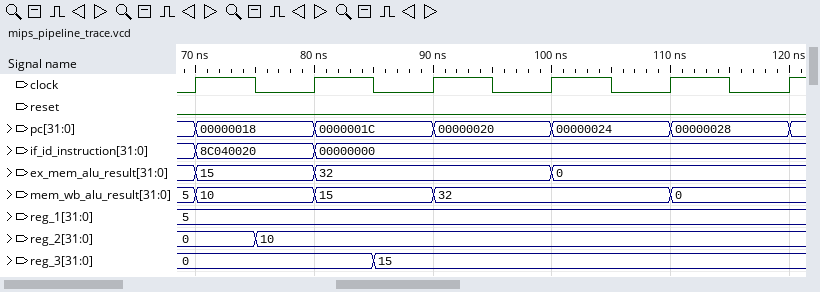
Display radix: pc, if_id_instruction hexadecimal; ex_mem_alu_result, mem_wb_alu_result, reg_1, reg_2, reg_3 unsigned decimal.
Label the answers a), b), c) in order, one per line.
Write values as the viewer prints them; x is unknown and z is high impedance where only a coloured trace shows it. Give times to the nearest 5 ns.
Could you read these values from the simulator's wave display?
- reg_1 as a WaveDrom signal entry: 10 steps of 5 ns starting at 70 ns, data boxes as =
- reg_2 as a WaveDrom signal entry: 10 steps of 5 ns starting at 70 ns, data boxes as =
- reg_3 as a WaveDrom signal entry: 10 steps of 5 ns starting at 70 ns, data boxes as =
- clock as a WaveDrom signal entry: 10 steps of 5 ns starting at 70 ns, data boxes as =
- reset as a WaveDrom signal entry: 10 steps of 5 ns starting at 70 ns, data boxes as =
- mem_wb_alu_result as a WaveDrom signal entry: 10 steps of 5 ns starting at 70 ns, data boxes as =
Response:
a) {name: 'reg_1', wave: '=.........', data: '5'}
b) {name: 'reg_2', wave: '==........', data: '0 10'}
c) {name: 'reg_3', wave: '=..=......', data: '0 15'}
d) {name: 'clock', wave: '1010101010'}
e) {name: 'reset', wave: '0.........'}
f) {name: 'mem_wb_alu_result', wave: '=.=.=...=.', data: '10 15 32 0'}
